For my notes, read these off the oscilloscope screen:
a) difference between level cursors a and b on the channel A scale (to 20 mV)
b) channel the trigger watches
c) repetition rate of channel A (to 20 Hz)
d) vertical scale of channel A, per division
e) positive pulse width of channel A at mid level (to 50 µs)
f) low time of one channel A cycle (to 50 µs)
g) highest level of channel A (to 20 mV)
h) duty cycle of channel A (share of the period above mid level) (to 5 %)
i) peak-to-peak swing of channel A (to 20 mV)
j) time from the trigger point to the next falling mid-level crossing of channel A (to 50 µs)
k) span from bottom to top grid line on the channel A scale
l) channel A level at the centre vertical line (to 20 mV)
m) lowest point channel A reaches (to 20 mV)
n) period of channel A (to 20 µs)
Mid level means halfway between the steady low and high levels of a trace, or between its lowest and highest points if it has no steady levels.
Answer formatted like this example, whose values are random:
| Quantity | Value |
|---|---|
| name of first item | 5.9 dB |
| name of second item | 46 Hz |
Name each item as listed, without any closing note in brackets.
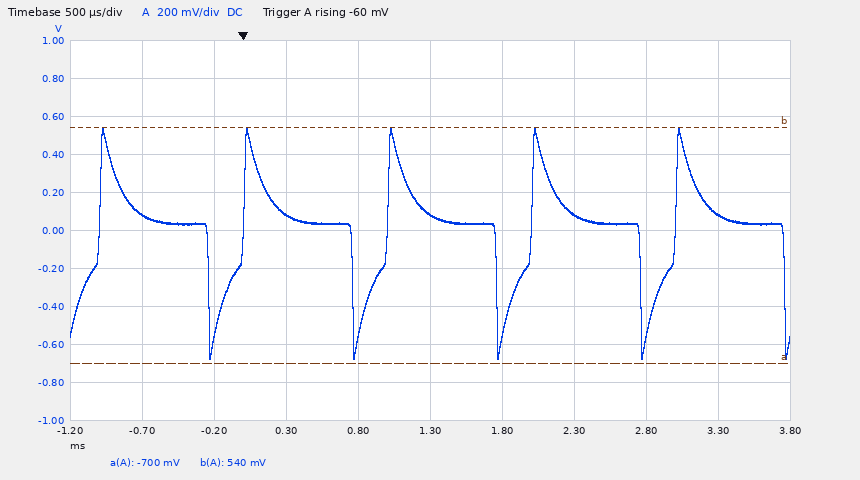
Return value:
| Quantity | Value |
|---|---|
| difference between level cursors a and b on the channel A scale | 1.24 V |
| channel the trigger watches | channel A |
| repetition rate of channel A | 1.00 kHz |
| vertical scale of channel A, per division | 200 mV |
| positive pulse width of channel A at mid level | 750 µs |
| low time of one channel A cycle | 250 µs |
| highest level of channel A | 540 mV |
| duty cycle of channel A (share of the period above mid level) | 75 % |
| peak-to-peak swing of channel A | 1.22 V |
| time from the trigger point to the next falling mid-level crossing of channel A | 750 µs |
| span from bottom to top grid line on the channel A scale | 2 V |
| channel A level at the centre vertical line | 80 mV |
| lowest point channel A reaches | -680 mV |
| period of channel A | 1.00 ms |
